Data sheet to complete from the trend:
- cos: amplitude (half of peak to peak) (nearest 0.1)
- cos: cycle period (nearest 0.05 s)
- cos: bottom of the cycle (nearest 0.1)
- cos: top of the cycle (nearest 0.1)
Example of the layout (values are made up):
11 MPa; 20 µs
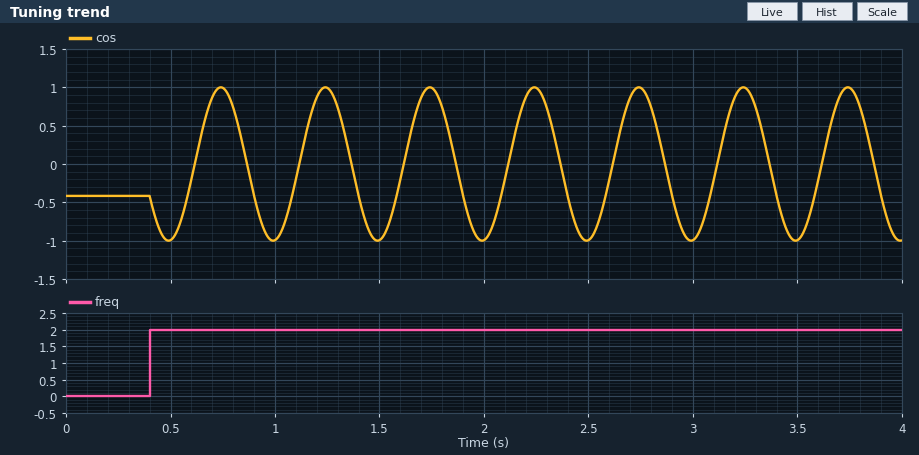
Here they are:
1.0; 0.50 s; -1.0; 1.0
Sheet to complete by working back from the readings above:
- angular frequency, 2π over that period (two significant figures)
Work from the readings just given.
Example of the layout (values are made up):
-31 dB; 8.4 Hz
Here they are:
13 rad/s
